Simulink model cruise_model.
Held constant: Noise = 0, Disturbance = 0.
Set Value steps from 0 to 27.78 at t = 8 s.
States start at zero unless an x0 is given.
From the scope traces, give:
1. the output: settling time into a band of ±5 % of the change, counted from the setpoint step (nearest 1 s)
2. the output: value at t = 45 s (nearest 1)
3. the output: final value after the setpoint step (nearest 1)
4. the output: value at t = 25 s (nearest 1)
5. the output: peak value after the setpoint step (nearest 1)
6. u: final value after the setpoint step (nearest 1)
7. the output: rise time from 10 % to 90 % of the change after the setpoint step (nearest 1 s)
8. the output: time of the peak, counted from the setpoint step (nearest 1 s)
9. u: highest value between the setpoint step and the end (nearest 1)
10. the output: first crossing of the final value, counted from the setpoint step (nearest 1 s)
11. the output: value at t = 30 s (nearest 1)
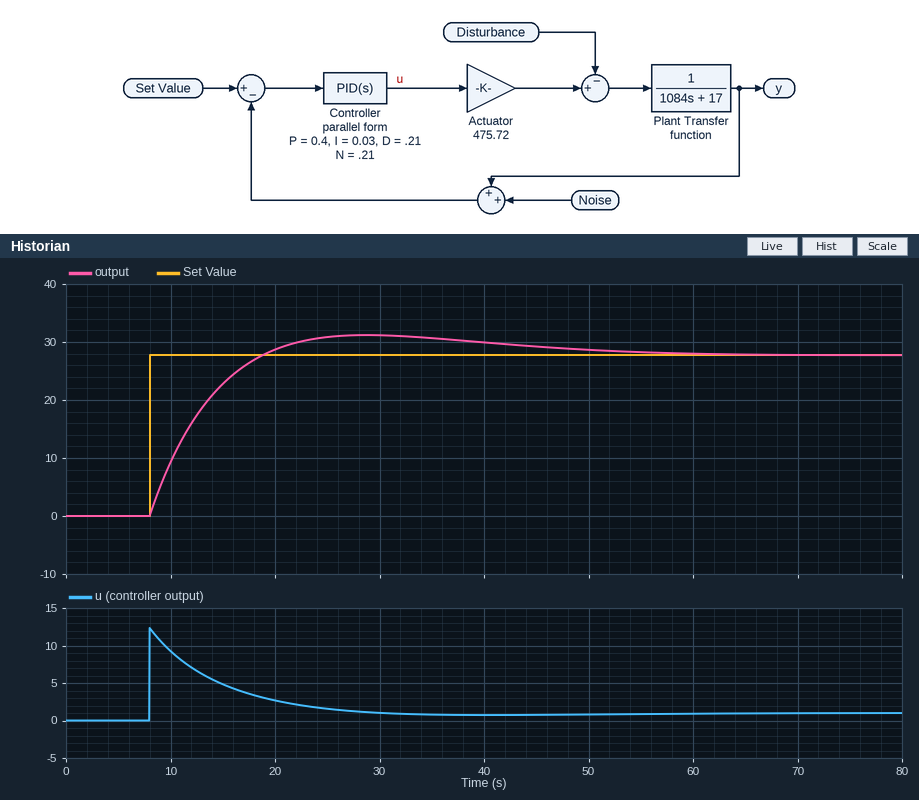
37 s
29
28
31
31
1
8 s
21 s
12
11 s
31
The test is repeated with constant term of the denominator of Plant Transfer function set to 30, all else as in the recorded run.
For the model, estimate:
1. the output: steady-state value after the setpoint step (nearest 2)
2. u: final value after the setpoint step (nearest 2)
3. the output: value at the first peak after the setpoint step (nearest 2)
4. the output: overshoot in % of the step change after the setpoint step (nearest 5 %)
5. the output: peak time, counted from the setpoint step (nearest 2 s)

28
2
30
10 %
22 s
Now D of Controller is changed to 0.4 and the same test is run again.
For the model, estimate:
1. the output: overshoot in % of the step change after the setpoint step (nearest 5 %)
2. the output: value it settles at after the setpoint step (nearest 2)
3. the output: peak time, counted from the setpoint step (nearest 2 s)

10 %
28
22 s
